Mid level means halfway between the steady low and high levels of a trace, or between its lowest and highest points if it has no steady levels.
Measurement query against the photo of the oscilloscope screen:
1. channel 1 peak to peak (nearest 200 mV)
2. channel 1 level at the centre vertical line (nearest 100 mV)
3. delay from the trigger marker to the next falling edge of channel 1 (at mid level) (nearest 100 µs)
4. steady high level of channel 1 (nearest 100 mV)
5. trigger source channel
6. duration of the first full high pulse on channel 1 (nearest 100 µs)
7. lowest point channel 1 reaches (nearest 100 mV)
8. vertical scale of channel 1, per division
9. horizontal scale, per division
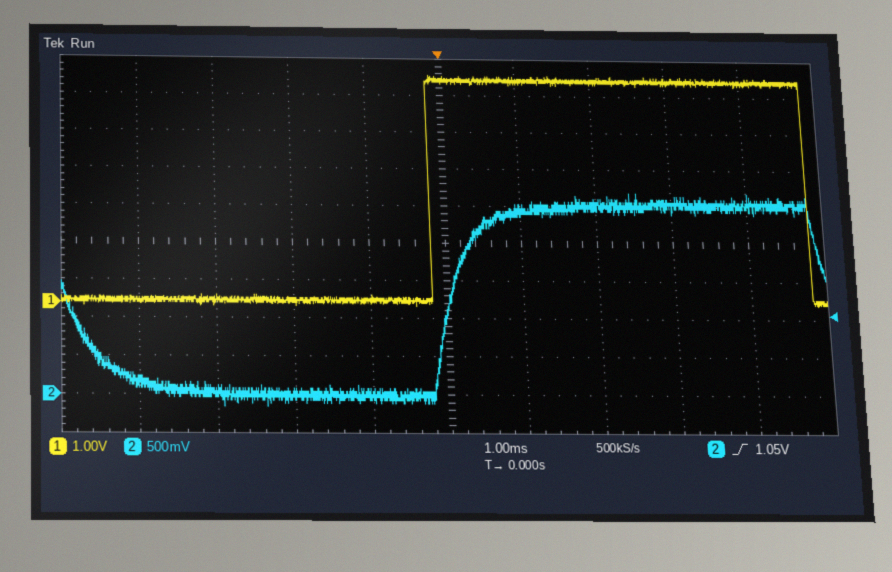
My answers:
6.2 V
6.0 V
4.8 ms
6.0 V
channel 2
5.0 ms
-100 mV
1 V
1 ms
